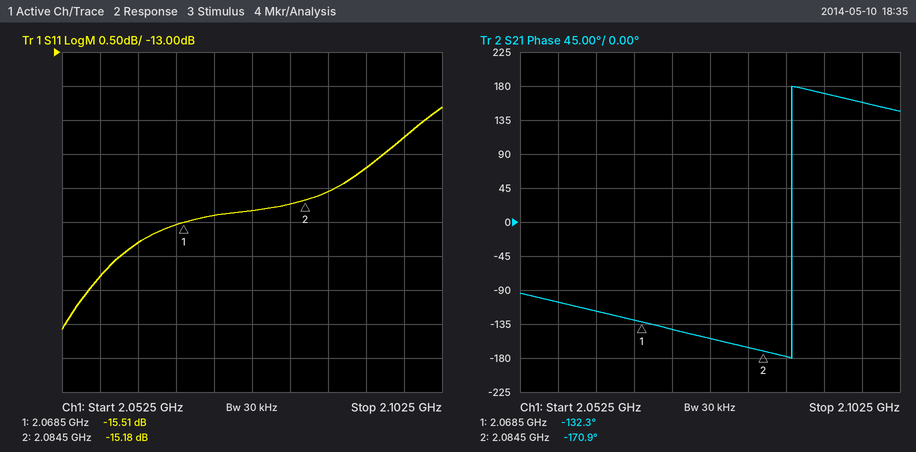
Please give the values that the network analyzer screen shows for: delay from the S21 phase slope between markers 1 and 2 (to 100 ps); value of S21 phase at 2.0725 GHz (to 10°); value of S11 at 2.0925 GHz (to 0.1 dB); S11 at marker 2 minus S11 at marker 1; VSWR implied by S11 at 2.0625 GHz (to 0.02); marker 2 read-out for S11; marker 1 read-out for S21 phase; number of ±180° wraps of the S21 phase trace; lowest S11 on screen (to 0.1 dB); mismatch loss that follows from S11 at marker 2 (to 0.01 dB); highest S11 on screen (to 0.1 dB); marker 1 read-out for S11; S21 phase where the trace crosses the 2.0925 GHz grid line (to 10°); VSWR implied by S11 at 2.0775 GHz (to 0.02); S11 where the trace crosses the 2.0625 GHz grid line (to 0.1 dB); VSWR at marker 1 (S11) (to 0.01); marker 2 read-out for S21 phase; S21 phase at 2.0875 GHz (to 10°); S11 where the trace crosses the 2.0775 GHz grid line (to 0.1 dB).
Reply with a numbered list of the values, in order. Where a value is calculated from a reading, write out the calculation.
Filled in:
1. −(-170.9° − (-132.3°))/(360° × 16 MHz) ≈ 6.7 ns
2. -140°
3. -14.7 dB
4. -15.18 − (-15.51) = 0.33 dB
5. |Γ| = 10^(-15.8/20) = 0.1622; VSWR = (1 + 0.1622)/(1 − 0.1622) ≈ 1.39, so 1.38 to the nearest 0.02
6. -15.18 dB
7. -132.3°
8. 1
9. -17.1 dB
10. −10 log10(1 − 10^(-15.18/10)) ≈ 0.13 dB
11. -13.8 dB
12. -15.51 dB
13. 170°
14. |Γ| = 10^(-15.3/20) = 0.1718; VSWR = (1 + 0.1718)/(1 − 0.1718) ≈ 1.41, so 1.42 to the nearest 0.02
15. -15.8 dB
16. (1 + 0.1677)/(1 − 0.1677) ≈ 1.40
17. -170.9°
18. -180°
19. -15.3 dB
